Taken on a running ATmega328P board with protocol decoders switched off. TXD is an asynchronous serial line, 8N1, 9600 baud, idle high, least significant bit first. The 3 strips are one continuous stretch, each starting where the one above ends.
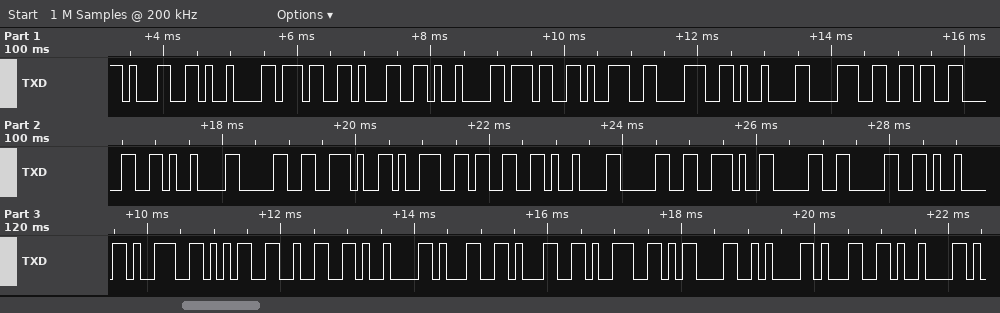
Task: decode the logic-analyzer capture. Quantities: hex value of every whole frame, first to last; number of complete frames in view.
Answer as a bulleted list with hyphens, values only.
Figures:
- 31 09 37 31 09 37 39 38 09 38 36 30 09 30 2E 39 33 09 30 2E 30 30 09 39 35 32 09 31 31 39 0D 0A 31 09
- 34
